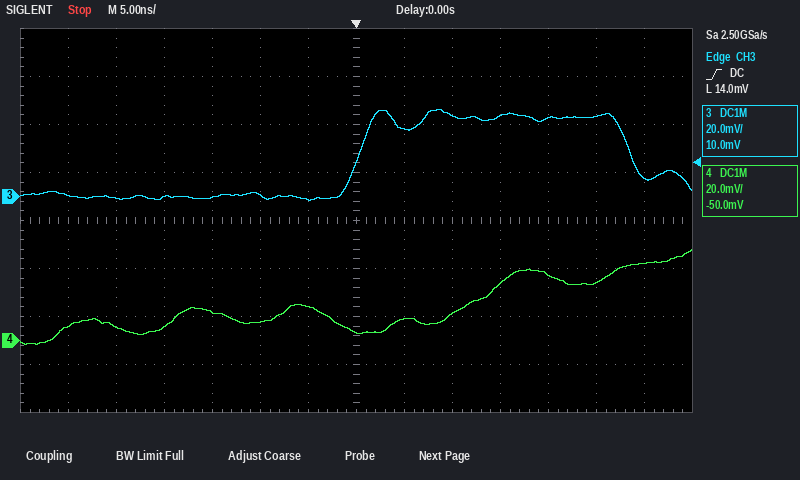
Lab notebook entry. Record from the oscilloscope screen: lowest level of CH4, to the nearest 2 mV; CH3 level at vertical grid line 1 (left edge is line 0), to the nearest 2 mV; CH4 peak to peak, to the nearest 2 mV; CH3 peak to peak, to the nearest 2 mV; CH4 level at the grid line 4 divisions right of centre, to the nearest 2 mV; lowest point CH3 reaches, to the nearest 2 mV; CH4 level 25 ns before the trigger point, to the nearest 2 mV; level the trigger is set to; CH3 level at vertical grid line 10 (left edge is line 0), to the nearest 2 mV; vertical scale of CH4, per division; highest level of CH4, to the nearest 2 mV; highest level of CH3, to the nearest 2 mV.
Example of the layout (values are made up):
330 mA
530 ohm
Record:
-2 mV
0 mV
40 mV
38 mV
28 mV
-2 mV
6 mV
14.0 mV
34 mV
20 mV
38 mV
36 mV
